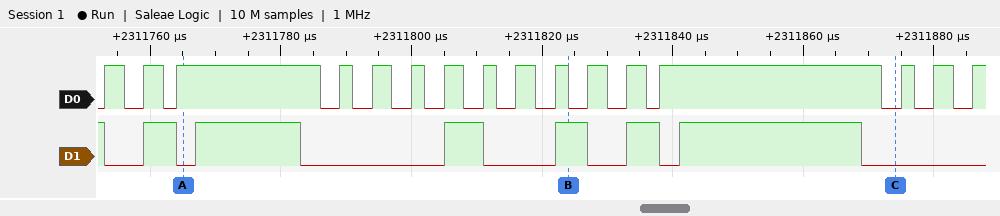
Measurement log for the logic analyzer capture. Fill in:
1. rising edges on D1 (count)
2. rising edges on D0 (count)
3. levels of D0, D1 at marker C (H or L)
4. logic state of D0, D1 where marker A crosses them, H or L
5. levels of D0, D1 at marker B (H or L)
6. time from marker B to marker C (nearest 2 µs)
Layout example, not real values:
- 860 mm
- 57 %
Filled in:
- 6
- 16
- D0=L, D1=L
- D0=H, D1=L
- D0=L, D1=H
- 50 µs
